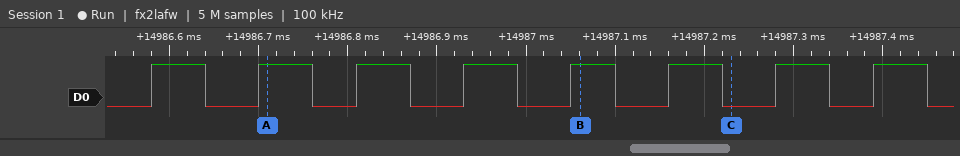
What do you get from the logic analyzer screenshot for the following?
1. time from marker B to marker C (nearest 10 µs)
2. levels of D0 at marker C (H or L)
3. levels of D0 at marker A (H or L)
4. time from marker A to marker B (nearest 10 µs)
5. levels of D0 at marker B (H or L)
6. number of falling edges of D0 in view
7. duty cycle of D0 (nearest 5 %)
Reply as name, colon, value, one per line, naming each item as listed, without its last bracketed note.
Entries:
time from marker B to marker C: 170 µs
levels of D0 at marker C: D0=L
levels of D0 at marker A: D0=H
time from marker A to marker B: 350 µs
levels of D0 at marker B: D0=H
number of falling edges of D0 in view: 8
duty cycle of D0: 50 %
